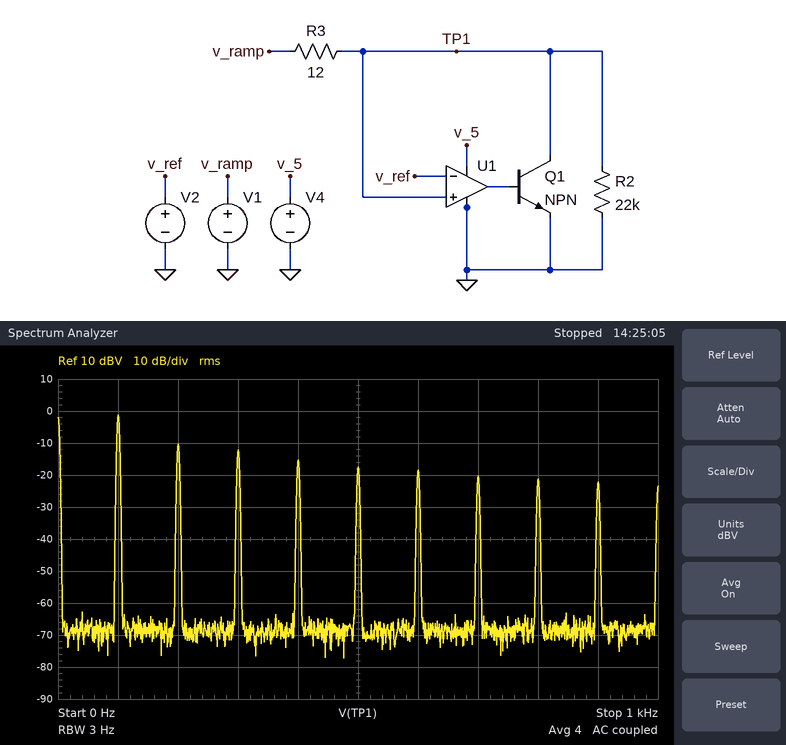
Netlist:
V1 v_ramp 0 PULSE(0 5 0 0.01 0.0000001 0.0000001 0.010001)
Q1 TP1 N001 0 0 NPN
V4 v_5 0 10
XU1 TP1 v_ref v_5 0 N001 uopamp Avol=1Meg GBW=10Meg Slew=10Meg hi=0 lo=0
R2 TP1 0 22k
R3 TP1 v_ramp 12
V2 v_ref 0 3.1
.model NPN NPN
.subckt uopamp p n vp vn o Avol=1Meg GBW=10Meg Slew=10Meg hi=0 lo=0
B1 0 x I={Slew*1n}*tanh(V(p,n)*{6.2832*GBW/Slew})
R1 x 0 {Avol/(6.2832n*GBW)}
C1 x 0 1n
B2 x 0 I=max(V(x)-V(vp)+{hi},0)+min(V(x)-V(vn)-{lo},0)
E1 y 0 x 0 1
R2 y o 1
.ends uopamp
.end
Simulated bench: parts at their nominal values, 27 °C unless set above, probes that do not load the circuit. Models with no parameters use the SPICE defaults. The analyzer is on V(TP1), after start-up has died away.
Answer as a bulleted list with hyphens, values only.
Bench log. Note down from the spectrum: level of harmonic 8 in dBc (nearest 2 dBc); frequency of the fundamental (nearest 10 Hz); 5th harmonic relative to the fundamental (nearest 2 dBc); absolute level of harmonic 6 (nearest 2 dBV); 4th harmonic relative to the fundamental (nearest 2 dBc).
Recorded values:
- -20 dBc
- 100 Hz
- -16 dBc
- -18 dBV
- -14 dBc
